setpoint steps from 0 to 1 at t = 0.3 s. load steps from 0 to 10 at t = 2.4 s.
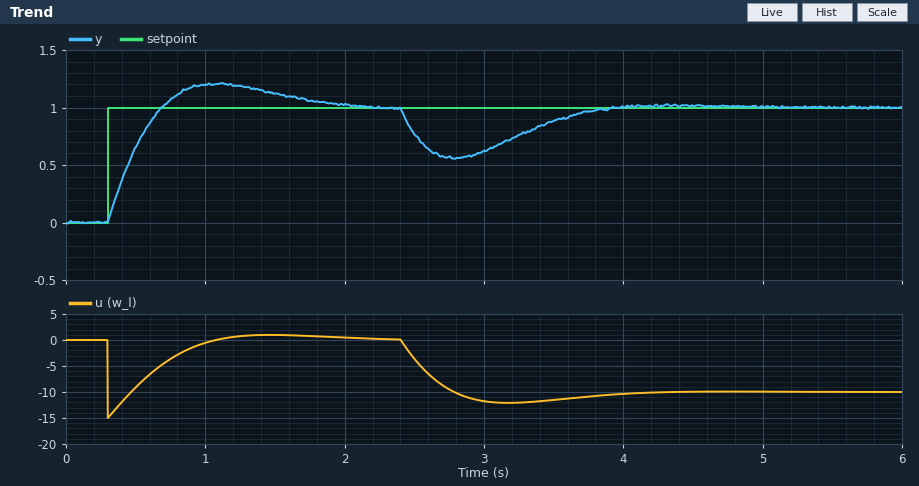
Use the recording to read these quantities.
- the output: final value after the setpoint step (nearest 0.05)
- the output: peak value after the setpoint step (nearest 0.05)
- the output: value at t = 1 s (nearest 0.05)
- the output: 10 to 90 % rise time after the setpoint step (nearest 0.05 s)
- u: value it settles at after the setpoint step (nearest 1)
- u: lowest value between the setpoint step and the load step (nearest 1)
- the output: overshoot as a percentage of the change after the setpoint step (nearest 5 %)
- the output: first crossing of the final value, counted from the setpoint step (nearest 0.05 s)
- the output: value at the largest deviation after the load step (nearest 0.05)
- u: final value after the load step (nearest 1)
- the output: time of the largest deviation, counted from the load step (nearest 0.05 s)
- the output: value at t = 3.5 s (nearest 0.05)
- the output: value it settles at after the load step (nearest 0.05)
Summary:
1.00
1.20
1.20
0.30 s
0
-15
20 %
0.40 s
0.55
-10
0.40 s
0.90
1.00
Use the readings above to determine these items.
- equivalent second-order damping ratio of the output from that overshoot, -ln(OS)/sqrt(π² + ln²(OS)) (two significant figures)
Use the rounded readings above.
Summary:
0.46
